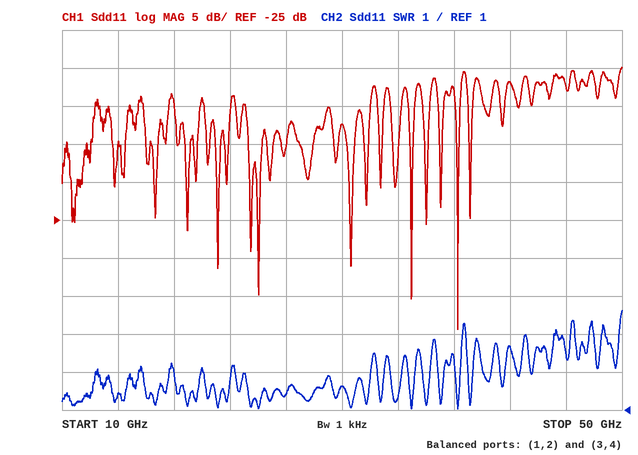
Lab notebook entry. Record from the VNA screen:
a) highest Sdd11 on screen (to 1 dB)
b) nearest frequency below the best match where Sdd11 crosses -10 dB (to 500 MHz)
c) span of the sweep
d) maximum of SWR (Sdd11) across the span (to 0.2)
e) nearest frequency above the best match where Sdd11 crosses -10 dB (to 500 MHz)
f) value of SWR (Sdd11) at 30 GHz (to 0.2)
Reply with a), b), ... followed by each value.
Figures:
a) -5 dB
b) 38.0 GHz
c) 40 GHz
d) 3.6
e) 38.5 GHz
f) 1.6
